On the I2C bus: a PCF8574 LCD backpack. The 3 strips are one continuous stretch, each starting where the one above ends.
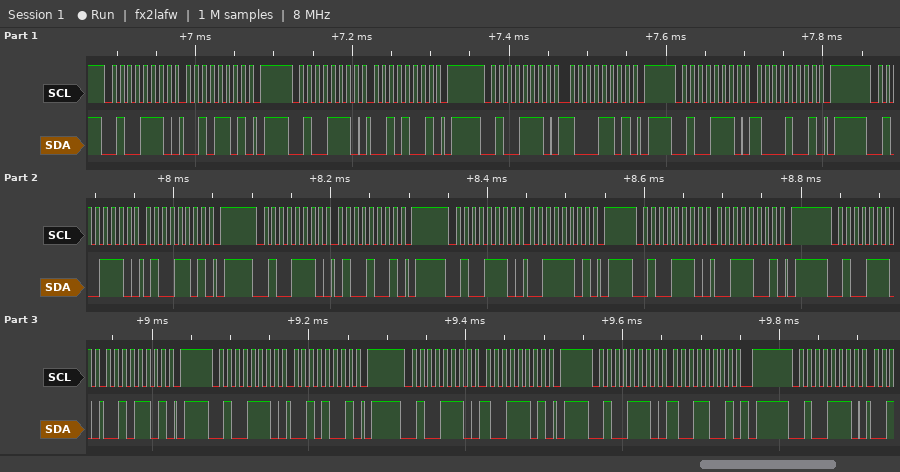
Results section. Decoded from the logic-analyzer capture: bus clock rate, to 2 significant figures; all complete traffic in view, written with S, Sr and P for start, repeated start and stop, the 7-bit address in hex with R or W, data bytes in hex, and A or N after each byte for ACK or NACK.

100 kHz
S 27W A 2D A P S 27W A 29 A P S 27W A 8D A P S 27W A 89 A P S 27W A 4D A P S 27W A 49 A P S 27W A 3D A P S 27W A 39 A P S 27W A 2D A P S 27W A 29 A P S 27W A 9D A P S 27W A 99 A P S 27W A
